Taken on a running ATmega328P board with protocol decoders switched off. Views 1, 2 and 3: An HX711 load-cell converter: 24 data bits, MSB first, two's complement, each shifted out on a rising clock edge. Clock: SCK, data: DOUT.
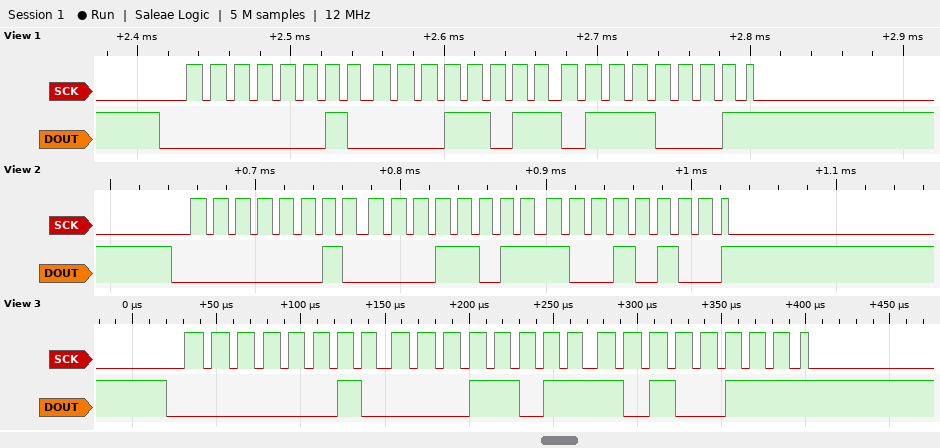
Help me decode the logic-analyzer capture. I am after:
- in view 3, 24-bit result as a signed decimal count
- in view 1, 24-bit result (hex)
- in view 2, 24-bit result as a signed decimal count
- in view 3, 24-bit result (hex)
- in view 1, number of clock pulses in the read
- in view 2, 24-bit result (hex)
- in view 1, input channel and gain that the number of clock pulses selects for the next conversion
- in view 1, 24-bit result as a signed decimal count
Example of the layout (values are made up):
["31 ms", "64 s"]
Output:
["138151", "0x021B71", "138132", "0x021BA7", "25", "0x021B94", "channel A, gain 128", "138097"]
